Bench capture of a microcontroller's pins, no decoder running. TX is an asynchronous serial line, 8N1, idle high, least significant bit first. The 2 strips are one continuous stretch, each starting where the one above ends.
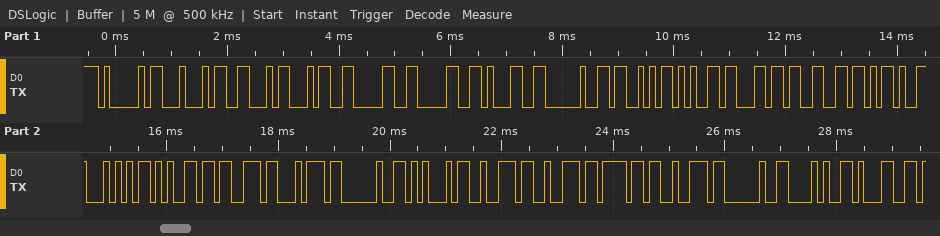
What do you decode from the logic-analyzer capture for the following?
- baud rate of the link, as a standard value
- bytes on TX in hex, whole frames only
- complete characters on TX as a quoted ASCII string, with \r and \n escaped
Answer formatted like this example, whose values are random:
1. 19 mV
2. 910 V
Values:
1. 9600 baud
2. 41 44 46 34 30 30 31 20 53 65 6C 66 2D 54 65 73 74 20 45 72 72 6F 72 20 28 31
3. "ADF4001 Self-Test Error (1"
